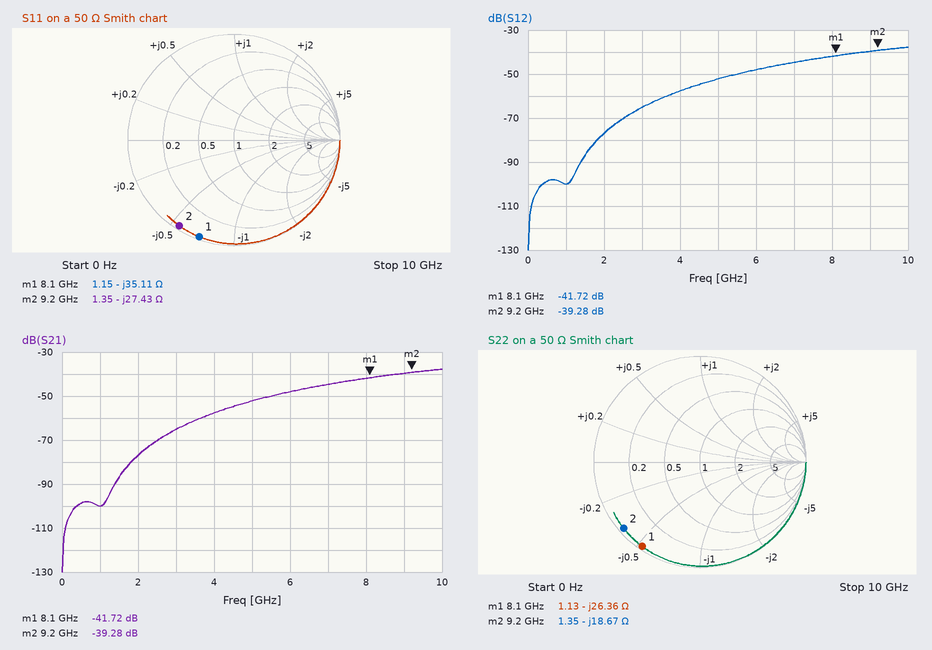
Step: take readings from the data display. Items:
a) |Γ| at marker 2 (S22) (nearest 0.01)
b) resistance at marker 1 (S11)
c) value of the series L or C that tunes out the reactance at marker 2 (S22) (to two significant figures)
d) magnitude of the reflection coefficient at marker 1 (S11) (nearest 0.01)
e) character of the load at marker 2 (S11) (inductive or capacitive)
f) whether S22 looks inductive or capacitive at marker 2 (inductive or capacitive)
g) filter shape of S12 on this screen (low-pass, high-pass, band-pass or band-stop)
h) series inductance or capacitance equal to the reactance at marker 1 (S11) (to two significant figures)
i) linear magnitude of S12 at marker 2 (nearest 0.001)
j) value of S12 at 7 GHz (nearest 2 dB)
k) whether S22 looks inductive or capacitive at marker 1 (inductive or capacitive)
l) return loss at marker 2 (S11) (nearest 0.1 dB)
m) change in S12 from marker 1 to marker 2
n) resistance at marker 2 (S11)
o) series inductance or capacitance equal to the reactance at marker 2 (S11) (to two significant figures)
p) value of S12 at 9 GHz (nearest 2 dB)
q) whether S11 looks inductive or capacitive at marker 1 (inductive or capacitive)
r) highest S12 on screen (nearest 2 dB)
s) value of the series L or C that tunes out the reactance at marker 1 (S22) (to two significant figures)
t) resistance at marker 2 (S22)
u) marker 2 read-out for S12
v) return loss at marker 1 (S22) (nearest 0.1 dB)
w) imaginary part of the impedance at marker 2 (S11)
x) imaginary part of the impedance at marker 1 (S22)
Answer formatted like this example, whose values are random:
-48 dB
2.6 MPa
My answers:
0.95
1.15 Ω
320 pH
0.97
capacitive
capacitive
high-pass
560 fF
0.011
-44 dB
capacitive
0.4 dB
2.44 dB
1.35 Ω
630 fF
-40 dB
capacitive
-38 dB
520 pH
1.35 Ω
-39.28 dB
0.3 dB
-27.43 Ω
-26.36 Ω
